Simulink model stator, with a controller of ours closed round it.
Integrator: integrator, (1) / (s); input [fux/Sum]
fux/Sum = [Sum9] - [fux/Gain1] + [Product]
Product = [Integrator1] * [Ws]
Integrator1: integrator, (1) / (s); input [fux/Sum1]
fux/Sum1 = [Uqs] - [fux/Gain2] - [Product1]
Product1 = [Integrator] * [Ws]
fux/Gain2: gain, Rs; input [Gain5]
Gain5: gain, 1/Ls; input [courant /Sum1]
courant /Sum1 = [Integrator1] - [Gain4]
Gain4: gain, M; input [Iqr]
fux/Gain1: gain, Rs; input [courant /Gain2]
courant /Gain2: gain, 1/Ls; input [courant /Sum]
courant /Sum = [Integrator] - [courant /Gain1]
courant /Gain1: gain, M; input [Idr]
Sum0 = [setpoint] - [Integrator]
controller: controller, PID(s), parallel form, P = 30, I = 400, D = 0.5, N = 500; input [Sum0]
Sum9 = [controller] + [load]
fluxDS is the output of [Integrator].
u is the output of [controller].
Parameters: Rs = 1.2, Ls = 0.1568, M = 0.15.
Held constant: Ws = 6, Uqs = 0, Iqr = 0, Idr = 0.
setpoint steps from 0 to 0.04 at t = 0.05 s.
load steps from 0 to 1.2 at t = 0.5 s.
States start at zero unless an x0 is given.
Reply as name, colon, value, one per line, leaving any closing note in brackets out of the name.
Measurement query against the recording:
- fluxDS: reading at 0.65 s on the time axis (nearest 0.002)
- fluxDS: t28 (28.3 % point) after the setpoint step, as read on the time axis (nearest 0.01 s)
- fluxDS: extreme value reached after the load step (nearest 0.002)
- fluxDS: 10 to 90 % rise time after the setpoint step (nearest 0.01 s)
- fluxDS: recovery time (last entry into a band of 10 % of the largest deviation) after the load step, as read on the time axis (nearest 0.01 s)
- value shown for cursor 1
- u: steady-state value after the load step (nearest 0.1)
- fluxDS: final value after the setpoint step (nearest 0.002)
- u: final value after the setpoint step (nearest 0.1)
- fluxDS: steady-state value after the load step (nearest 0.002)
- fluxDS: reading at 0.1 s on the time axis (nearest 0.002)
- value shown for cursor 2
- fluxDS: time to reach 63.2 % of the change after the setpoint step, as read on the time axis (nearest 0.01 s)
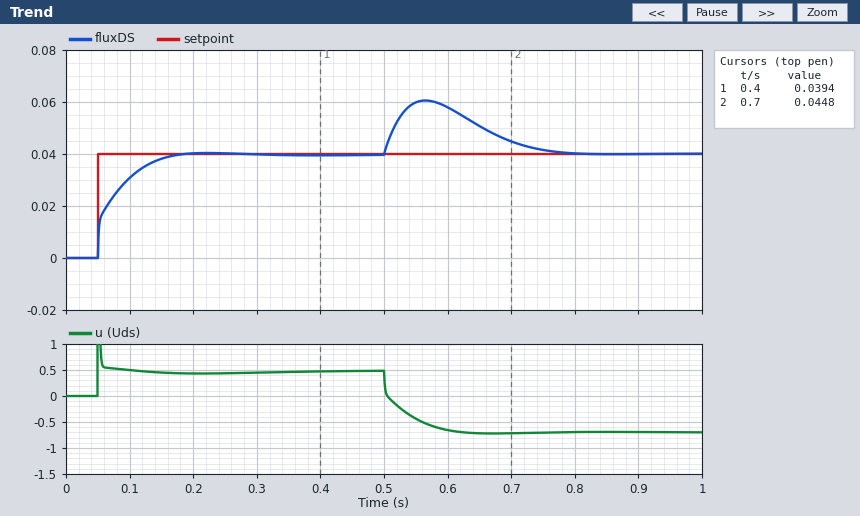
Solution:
fluxDS: reading at 0.65 s on the time axis: 0.050
fluxDS: t28 (28.3 % point) after the setpoint step, as read on the time axis: 0.05 s
fluxDS: extreme value reached after the load step: 0.060
fluxDS: 10 to 90 % rise time after the setpoint step: 0.08 s
fluxDS: recovery time (last entry into a band of 10 % of the largest deviation) after the load step, as read on the time axis: 0.74 s
value shown for cursor 1: 0.0394
u: steady-state value after the load step: -0.7
fluxDS: final value after the setpoint step: 0.040
u: final value after the setpoint step: 0.5
fluxDS: steady-state value after the load step: 0.040
fluxDS: reading at 0.1 s on the time axis: 0.030
value shown for cursor 2: 0.0448
fluxDS: time to reach 63.2 % of the change after the setpoint step, as read on the time axis: 0.08 s
